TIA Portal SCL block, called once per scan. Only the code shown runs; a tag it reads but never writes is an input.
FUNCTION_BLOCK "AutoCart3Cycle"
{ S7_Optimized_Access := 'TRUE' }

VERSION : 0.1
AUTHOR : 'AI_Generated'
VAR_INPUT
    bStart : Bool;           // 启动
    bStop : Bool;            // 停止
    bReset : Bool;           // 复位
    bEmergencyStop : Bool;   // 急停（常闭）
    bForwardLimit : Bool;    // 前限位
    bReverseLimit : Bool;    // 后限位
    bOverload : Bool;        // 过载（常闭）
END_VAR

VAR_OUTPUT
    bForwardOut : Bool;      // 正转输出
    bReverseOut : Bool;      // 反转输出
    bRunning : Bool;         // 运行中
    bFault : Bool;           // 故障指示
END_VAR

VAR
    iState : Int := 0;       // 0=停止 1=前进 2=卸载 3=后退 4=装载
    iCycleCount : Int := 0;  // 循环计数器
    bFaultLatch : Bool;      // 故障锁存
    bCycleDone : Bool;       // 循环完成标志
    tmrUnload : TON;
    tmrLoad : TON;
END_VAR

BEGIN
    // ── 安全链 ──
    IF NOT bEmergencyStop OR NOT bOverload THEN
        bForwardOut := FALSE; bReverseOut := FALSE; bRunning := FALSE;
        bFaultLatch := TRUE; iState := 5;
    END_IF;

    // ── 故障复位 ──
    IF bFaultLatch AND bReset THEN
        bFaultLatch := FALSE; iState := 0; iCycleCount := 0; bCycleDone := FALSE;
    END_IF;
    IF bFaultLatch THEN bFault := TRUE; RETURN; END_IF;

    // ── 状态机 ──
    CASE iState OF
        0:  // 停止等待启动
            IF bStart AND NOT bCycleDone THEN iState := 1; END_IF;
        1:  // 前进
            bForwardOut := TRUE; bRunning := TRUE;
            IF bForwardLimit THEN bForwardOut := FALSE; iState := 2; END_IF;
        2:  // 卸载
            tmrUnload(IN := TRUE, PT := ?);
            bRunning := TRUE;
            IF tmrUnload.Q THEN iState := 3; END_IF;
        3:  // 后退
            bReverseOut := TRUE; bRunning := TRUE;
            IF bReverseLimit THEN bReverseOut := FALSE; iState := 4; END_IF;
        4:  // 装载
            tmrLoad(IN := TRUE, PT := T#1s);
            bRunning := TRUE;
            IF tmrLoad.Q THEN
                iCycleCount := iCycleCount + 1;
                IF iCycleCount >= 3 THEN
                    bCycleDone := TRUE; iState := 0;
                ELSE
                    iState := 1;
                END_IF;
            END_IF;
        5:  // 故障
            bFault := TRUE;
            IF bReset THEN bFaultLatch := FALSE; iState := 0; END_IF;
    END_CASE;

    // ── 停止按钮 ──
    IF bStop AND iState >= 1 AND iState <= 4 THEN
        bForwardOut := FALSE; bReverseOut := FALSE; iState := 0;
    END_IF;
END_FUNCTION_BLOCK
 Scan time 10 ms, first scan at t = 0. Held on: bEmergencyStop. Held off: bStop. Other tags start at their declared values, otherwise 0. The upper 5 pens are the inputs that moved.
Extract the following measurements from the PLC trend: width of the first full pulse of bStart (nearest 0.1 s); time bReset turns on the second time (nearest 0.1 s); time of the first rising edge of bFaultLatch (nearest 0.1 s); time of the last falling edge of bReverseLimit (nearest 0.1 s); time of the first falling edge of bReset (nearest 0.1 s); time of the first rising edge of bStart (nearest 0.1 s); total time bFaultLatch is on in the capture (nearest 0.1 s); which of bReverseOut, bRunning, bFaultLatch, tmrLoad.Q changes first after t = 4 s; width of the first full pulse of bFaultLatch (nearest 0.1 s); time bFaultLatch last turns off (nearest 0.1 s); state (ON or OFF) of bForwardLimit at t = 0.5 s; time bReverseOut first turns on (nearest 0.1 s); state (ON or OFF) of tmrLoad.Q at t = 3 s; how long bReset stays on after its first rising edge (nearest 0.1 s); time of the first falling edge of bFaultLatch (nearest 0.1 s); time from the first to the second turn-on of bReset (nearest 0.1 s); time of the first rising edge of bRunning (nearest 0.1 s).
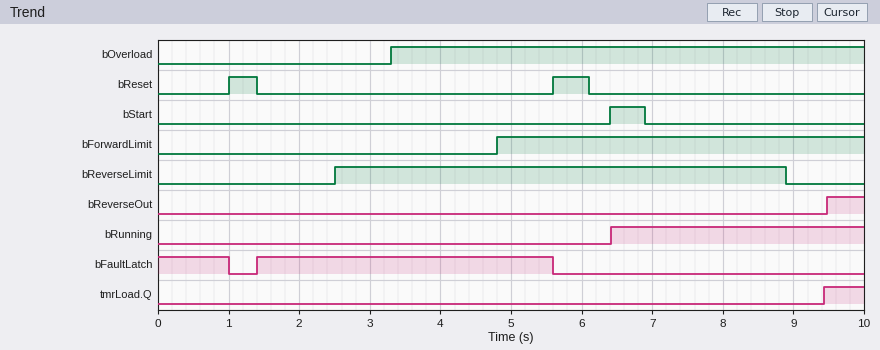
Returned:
0.5 s
5.6 s
1.4 s
8.9 s
1.4 s
6.4 s
5.2 s
bFaultLatch
4.2 s
5.6 s
OFF
9.5 s
OFF
0.4 s
1.0 s
4.6 s
6.4 s
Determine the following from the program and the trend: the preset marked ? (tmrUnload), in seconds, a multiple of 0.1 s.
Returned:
2.0 s
